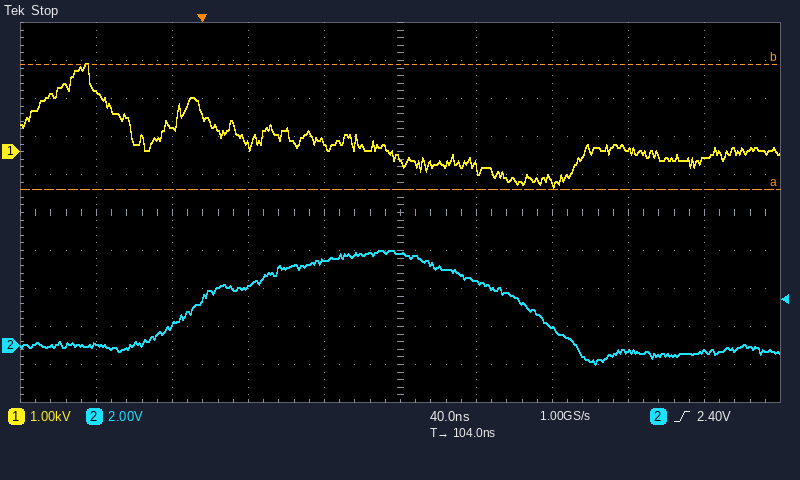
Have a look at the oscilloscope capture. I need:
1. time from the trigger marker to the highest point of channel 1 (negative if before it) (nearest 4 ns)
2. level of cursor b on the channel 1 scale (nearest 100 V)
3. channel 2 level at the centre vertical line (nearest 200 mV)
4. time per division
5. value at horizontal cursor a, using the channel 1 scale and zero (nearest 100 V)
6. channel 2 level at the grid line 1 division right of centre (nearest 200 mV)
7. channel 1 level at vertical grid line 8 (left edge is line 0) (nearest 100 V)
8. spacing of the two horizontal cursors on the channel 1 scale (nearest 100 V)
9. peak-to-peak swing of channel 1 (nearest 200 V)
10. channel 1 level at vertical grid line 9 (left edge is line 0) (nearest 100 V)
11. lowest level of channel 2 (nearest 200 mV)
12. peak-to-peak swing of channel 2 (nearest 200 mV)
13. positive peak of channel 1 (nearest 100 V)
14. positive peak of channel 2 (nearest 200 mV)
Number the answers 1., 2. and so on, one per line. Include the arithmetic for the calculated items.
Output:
1. -60 ns
2. 2.3 kV
3. 4.8 V
4. 40 ns
5. -1.0 kV
6. 3.4 V
7. 0.0 kV
8. 3.3 kV
9. 3.2 kV
10. -200 V
11. -1.0 V
12. 5.0 V − (-1.0 V) = 6.0 V
13. 2.3 kV
14. 5.0 V
